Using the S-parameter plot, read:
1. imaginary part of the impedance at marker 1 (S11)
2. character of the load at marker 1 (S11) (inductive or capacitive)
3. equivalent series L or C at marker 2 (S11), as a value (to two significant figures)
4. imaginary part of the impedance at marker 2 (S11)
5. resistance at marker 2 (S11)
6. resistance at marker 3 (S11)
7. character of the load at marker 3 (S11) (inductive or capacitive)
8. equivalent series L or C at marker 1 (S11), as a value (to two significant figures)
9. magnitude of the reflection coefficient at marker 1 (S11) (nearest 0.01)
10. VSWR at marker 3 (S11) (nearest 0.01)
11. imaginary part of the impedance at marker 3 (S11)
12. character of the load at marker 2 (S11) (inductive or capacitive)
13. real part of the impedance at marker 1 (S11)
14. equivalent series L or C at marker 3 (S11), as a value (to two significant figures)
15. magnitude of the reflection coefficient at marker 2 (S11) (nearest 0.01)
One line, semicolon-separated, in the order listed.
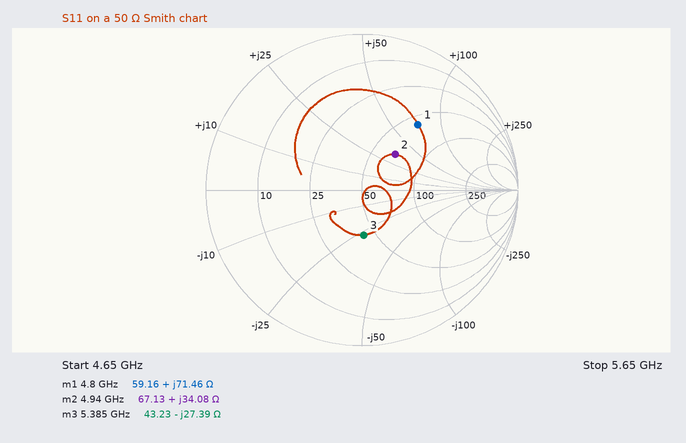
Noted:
+71.46 Ω; inductive; 1.1 nH; +34.08 Ω; 67.13 Ω; 43.23 Ω; capacitive; 2.4 nH; 0.55; 1.82; -27.39 Ω; inductive; 59.16 Ω; 1.1 pF; 0.31
